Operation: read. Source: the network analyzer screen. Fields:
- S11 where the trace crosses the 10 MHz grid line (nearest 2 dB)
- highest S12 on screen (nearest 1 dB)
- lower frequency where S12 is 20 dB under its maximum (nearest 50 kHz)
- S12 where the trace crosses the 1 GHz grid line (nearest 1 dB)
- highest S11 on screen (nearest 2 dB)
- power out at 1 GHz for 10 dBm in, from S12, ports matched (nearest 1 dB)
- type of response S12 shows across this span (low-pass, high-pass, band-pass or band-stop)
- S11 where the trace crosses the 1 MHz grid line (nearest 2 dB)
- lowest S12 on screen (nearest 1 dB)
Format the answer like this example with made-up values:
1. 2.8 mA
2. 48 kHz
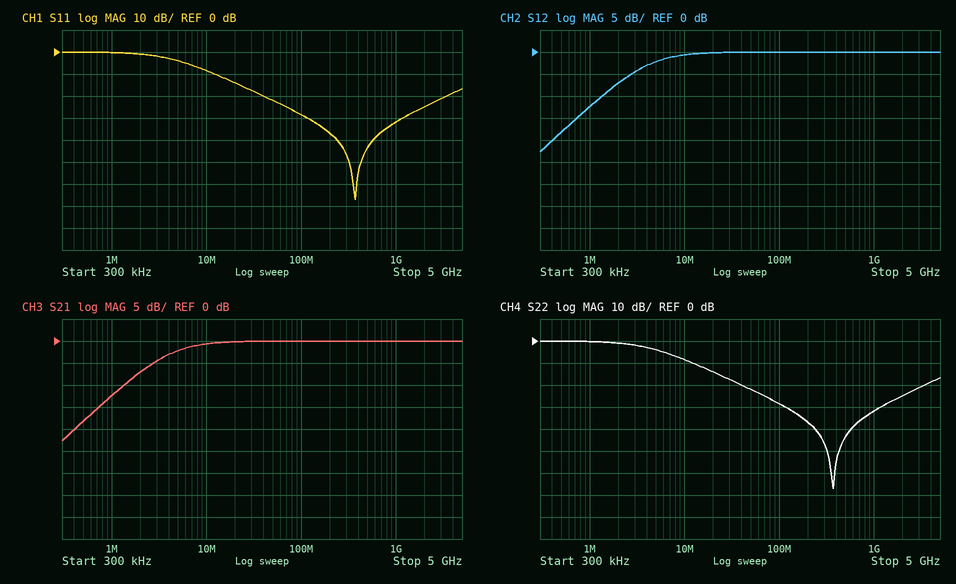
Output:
1. -8 dB
2. 0 dB
3. 400 kHz
4. 0 dB
5. 0 dB
6. 10 dBm
7. high-pass
8. 0 dB
9. -23 dB
